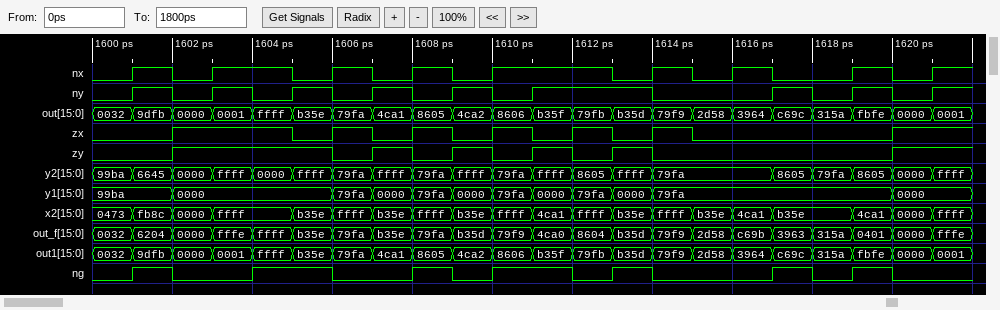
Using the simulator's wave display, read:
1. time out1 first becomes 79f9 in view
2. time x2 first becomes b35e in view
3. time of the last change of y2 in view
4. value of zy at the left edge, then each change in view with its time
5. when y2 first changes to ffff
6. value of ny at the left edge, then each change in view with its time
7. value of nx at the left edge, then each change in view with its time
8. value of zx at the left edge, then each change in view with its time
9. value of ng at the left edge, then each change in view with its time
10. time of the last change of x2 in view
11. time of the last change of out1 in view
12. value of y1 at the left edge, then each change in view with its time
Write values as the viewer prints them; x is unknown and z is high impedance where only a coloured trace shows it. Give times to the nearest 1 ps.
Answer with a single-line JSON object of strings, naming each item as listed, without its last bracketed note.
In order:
{"time out1 first becomes 79f9 in view": "1614 ps", "time x2 first becomes b35e in view": "1605 ps", "time of the last change of y2 in view": "1621 ps", "value of zy at the left edge, then each change in view with its time": "0, 1 at 1602 ps, 0 at 1606 ps, 1 at 1607 ps, 0 at 1608 ps, 1 at 1609 ps, 0 at 1610 ps, 1 at 1611 ps, 0 at 1612 ps, 1 at 1613 ps, 0 at 1614 ps, 1 at 1620 ps", "when y2 first changes to ffff": "1603 ps", "value of ny at the left edge, then each change in view with its time": "0, 1 at 1601 ps, 0 at 1602 ps, 1 at 1603 ps, 0 at 1604 ps, 1 at 1605 ps, 0 at 1606 ps, 1 at 1607 ps, 0 at 1608 ps, 1 at 1609 ps, 0 at 1610 ps, 1 at 1611 ps, 0 at 1614 ps, 1 at 1617 ps, 0 at 1618 ps, 1 at 1619 ps, 0 at 1620 ps, 1 at 1621 ps", "value of nx at the left edge, then each change in view with its time": "0, 1 at 1601 ps, 0 at 1602 ps, 1 at 1603 ps, 0 at 1605 ps, 1 at 1606 ps, 0 at 1607 ps, 1 at 1608 ps, 0 at 1609 ps, 1 at 1610 ps, 0 at 1613 ps, 1 at 1614 ps, 0 at 1615 ps, 1 at 1616 ps, 0 at 1617 ps, 1 at 1619 ps, 0 at 1620 ps, 1 at 1621 ps", "value of zx at the left edge, then each change in view with its time": "0, 1 at 1602 ps, 0 at 1605 ps, 1 at 1606 ps, 0 at 1607 ps, 1 at 1608 ps, 0 at 1609 ps, 1 at 1610 ps, 0 at 1611 ps, 1 at 1612 ps, 0 at 1613 ps, 1 at 1614 ps, 0 at 1615 ps, 1 at 1620 ps", "value of ng at the left edge, then each change in view with its time": "0, 1 at 1601 ps, 0 at 1602 ps, 1 at 1604 ps, 0 at 1606 ps, 1 at 1608 ps, 0 at 1609 ps, 1 at 1610 ps, 0 at 1612 ps, 1 at 1613 ps, 0 at 1614 ps, 1 at 1617 ps, 0 at 1618 ps, 1 at 1619 ps, 0 at 1620 ps", "time of the last change of x2 in view": "1621 ps", "time of the last change of out1 in view": "1621 ps", "value of y1 at the left edge, then each change in view with its time": "99ba, 0000 at 1602 ps, 79fa at 1606 ps, 0000 at 1607 ps, 79fa at 1608 ps, 0000 at 1609 ps, 79fa at 1610 ps, 0000 at 1611 ps, 79fa at 1612 ps, 0000 at 1613 ps, 79fa at 1614 ps, 0000 at 1620 ps"}
